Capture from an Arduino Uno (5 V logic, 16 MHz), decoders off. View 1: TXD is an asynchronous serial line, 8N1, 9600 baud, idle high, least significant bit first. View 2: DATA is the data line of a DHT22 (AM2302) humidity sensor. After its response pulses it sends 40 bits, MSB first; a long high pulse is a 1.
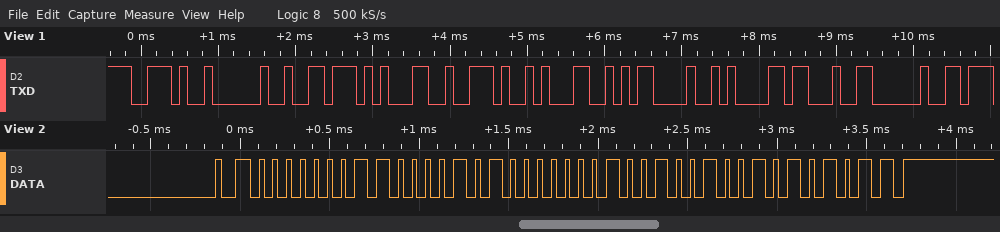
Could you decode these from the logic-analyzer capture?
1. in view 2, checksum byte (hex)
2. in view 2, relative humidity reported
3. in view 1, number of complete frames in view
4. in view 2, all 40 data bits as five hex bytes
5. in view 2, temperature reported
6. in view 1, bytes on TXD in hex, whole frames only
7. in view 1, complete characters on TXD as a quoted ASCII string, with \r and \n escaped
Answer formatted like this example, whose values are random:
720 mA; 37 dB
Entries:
0xAB; 38.9 %; 10; 01 85 01 24 AB; 29.2 °C; 0x2E 0x20 0x76 0x31 0x2E 0x31 0x0D 0x0A 0x23 0x20; ". v1.1\r\n# "
